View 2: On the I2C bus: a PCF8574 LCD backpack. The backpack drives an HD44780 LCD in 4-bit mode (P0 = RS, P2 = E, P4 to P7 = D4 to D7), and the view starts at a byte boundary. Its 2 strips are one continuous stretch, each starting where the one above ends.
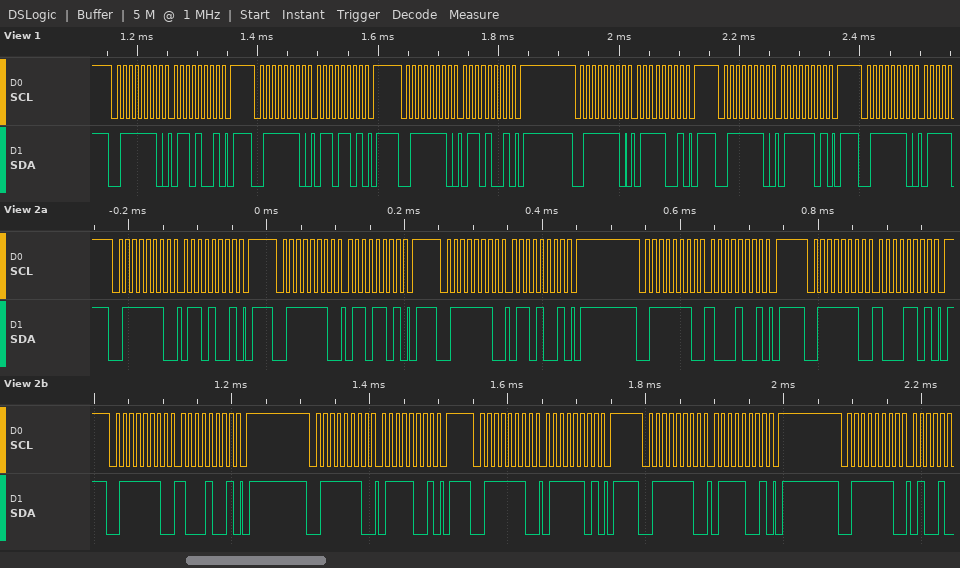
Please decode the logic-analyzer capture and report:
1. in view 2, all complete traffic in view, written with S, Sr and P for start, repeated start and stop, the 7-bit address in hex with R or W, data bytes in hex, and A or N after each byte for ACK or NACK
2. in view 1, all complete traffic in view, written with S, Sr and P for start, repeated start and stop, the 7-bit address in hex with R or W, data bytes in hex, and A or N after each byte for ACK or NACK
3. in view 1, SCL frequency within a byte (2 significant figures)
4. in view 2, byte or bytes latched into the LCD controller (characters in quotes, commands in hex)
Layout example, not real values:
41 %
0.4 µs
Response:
S 3FW A 69 A P S 3FW A 6D A P S 3FW A 69 A P S 3FW A 89 A P S 3FW A 8D A P S 3FW A 89 A P S 3FW A 79 A P S 3FW A 7D A P S 3FW A 79 A P S 3FW A
S 3FW A 69 A P S 3FW A 6D A P S 3FW A 69 A P S 3FW A 79 A P S 3FW A 7D A P S 3FW A
100 kHz
'h'
